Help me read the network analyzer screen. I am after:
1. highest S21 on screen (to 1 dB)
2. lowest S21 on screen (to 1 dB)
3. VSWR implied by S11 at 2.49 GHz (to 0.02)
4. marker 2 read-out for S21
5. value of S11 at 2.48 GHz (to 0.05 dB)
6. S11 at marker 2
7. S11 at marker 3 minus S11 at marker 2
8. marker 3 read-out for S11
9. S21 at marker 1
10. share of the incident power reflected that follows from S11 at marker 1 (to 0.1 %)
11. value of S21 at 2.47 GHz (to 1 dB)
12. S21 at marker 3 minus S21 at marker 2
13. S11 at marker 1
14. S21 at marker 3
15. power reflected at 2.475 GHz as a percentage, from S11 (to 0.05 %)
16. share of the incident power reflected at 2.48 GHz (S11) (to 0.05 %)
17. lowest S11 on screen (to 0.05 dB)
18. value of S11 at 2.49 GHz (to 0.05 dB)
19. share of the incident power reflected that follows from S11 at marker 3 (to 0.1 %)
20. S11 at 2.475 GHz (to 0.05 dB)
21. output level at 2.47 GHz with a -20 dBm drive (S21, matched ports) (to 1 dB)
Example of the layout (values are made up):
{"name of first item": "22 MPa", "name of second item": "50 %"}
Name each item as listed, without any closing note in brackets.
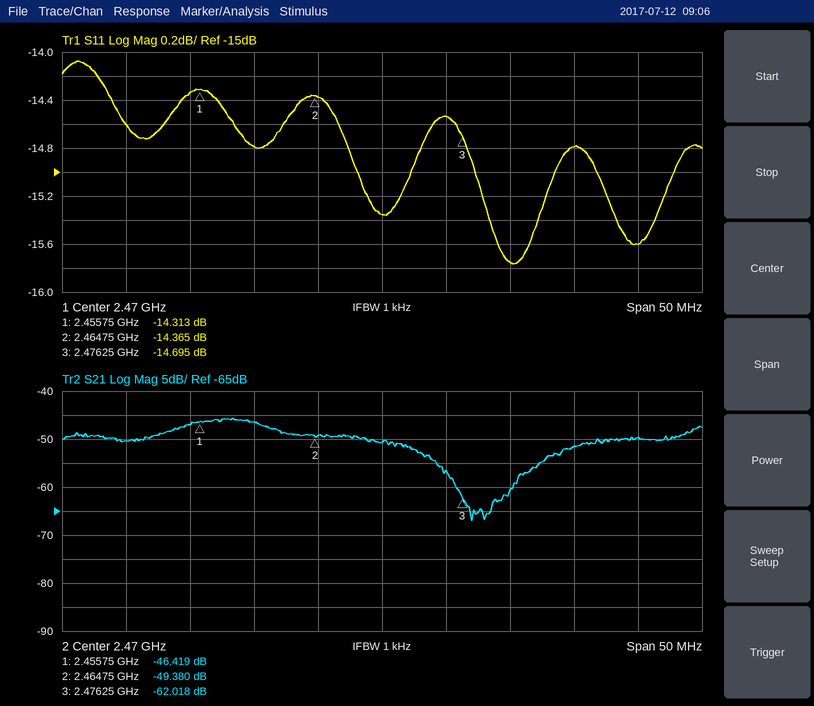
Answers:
{"highest S21 on screen": "-46 dB", "lowest S21 on screen": "-67 dB", "VSWR implied by S11 at 2.49 GHz": "1.40", "marker 2 read-out for S21": "-49.380 dB", "value of S11 at 2.48 GHz": "-15.75 dB", "S11 at marker 2": "-14.365 dB", "S11 at marker 3 minus S11 at marker 2": "-0.330 dB", "marker 3 read-out for S11": "-14.695 dB", "S21 at marker 1": "-46.419 dB", "share of the incident power reflected that follows from S11 at marker 1": "3.7 %", "value of S21 at 2.47 GHz": "-51 dB", "S21 at marker 3 minus S21 at marker 2": "-12.638 dB", "S11 at marker 1": "-14.313 dB", "S21 at marker 3": "-62.018 dB", "power reflected at 2.475 GHz as a percentage, from S11": "3.50 %", "share of the incident power reflected at 2.48 GHz (S11)": "2.65 %", "lowest S11 on screen": "-15.75 dB", "value of S11 at 2.49 GHz": "-15.60 dB", "share of the incident power reflected that follows from S11 at marker 3": "3.4 %", "S11 at 2.475 GHz": "-14.55 dB", "output level at 2.47 GHz with a -20 dBm drive (S21, matched ports)": "-71 dBm"}
